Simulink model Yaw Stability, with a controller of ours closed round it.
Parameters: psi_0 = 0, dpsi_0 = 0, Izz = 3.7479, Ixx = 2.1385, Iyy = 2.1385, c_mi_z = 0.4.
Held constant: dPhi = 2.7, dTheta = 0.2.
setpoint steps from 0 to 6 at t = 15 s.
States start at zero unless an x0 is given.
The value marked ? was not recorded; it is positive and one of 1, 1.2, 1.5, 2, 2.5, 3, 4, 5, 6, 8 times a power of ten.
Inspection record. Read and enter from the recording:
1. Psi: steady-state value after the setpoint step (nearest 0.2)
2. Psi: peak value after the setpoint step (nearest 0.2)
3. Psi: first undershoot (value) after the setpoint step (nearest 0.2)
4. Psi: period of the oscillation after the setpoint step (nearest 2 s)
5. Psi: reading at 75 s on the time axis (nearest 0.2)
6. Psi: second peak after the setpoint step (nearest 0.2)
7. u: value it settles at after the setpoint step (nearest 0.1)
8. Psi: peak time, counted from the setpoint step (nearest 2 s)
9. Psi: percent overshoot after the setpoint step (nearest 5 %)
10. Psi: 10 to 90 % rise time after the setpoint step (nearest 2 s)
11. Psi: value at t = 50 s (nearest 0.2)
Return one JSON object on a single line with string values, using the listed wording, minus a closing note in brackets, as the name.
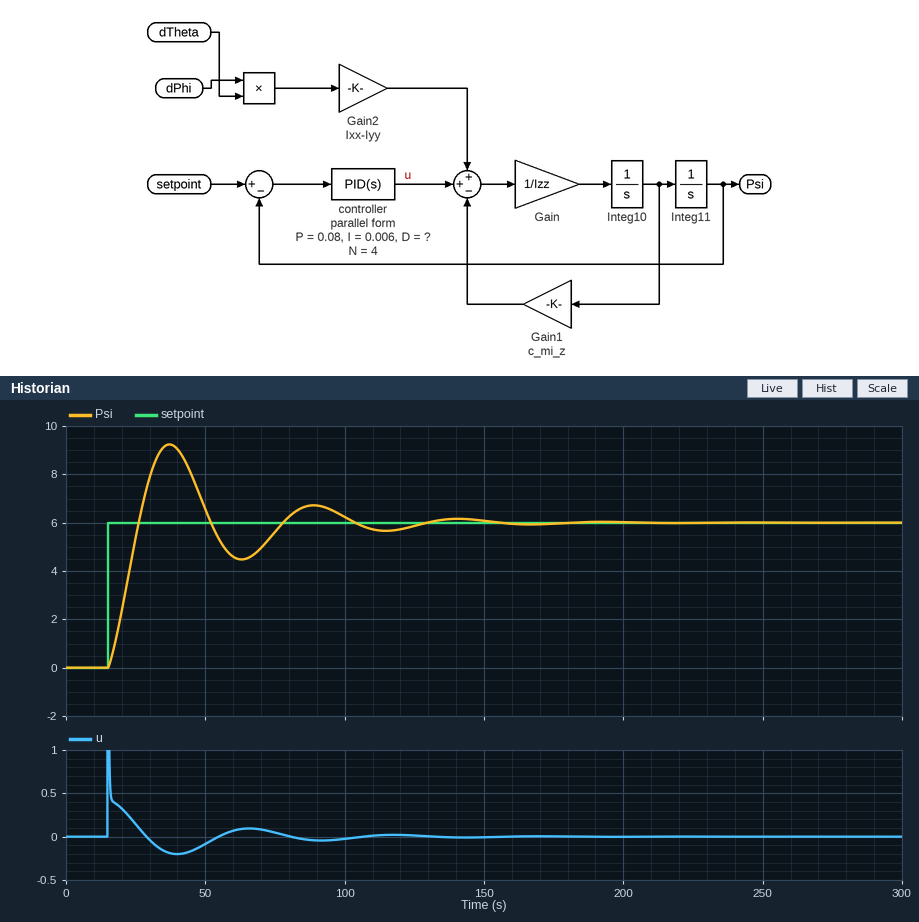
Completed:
{"Psi: steady-state value after the setpoint step": "6.0", "Psi: peak value after the setpoint step": "9.2", "Psi: first undershoot (value) after the setpoint step": "4.4", "Psi: period of the oscillation after the setpoint step": "52 s", "Psi: reading at 75 s on the time axis": "5.6", "Psi: second peak after the setpoint step": "6.8", "u: value it settles at after the setpoint step": "0.0", "Psi: peak time, counted from the setpoint step": "22 s", "Psi: percent overshoot after the setpoint step": "55 %", "Psi: 10 to 90 % rise time after the setpoint step": "8 s", "Psi: value at t = 50 s": "6.6"}
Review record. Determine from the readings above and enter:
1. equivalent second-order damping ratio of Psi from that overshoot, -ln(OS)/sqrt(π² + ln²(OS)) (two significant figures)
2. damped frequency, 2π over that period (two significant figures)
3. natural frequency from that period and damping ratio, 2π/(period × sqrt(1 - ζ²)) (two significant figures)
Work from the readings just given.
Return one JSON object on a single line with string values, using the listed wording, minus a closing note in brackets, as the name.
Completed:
{"equivalent second-order damping ratio of Psi from that overshoot, -ln(OS)/sqrt(π² + ln²(OS))": "0.19", "damped frequency, 2π over that period": "0.12 rad/s", "natural frequency from that period and damping ratio, 2π/(period × sqrt(1 - ζ²))": "0.12 rad/s"}
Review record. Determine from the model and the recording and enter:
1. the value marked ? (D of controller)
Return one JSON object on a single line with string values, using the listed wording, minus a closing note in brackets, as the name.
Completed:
{"the value marked ?": "0.2"}
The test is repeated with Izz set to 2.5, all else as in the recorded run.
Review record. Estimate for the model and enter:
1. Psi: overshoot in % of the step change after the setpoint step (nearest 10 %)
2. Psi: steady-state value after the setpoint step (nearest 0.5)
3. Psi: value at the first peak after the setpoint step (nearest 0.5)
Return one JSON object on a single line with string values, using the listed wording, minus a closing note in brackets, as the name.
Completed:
{"Psi: overshoot in % of the step change after the setpoint step": "40 %", "Psi: steady-state value after the setpoint step": "6.0", "Psi: value at the first peak after the setpoint step": "8.5"}
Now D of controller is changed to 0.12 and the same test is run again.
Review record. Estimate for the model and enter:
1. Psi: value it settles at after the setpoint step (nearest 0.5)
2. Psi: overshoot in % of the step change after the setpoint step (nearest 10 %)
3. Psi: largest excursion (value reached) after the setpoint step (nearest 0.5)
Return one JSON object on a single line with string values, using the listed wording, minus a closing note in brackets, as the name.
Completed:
{"Psi: value it settles at after the setpoint step": "6.0", "Psi: overshoot in % of the step change after the setpoint step": "60 %", "Psi: largest excursion (value reached) after the setpoint step": "10.0"}
